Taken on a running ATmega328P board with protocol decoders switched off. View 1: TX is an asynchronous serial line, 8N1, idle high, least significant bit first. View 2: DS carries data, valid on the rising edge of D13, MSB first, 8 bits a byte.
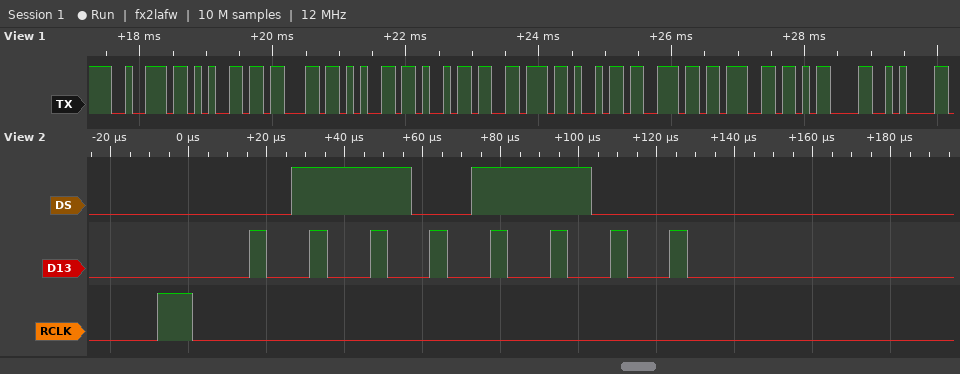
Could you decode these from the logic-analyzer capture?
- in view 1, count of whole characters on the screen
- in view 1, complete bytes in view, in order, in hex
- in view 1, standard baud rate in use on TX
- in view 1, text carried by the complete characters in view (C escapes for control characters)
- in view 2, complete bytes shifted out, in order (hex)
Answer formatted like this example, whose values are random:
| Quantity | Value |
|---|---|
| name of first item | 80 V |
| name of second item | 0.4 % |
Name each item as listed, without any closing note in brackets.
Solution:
| Quantity | Value |
|---|---|
| in view 1, count of whole characters on the screen | 11 |
| in view 1, complete bytes in view, in order, in hex | 72 65 63 65 69 76 69 6E 67 0D 0A |
| in view 1, standard baud rate in use on TX | 9600 baud |
| in view 1, text carried by the complete characters in view | "receiving\r\n" |
| in view 2, complete bytes shifted out, in order | 0x6C |
